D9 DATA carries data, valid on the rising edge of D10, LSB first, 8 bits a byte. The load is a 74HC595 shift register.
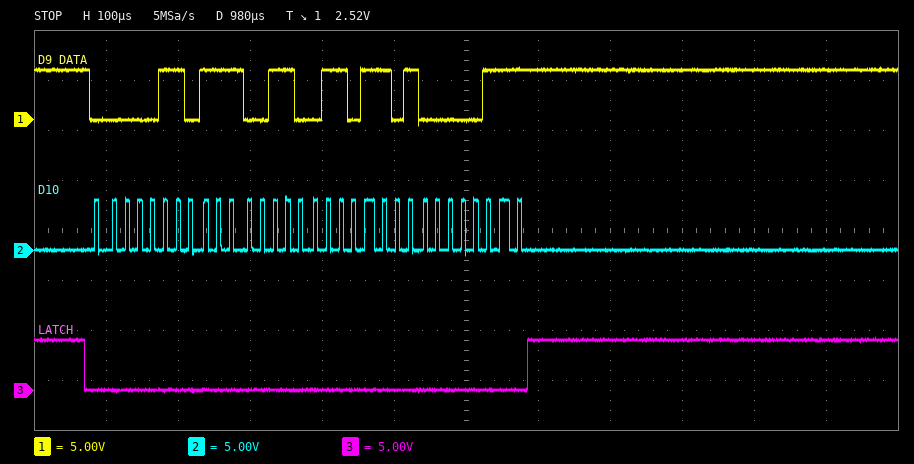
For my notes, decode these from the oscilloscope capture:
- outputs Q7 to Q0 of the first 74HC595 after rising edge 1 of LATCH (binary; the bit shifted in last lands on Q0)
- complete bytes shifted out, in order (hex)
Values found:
00000111
60 67 B6 E0
